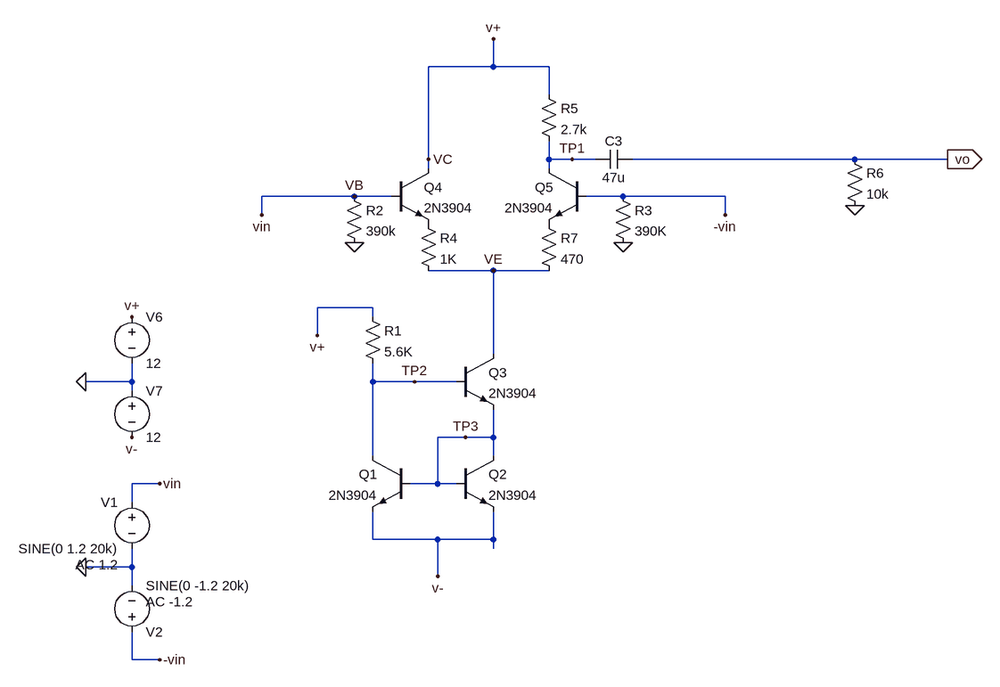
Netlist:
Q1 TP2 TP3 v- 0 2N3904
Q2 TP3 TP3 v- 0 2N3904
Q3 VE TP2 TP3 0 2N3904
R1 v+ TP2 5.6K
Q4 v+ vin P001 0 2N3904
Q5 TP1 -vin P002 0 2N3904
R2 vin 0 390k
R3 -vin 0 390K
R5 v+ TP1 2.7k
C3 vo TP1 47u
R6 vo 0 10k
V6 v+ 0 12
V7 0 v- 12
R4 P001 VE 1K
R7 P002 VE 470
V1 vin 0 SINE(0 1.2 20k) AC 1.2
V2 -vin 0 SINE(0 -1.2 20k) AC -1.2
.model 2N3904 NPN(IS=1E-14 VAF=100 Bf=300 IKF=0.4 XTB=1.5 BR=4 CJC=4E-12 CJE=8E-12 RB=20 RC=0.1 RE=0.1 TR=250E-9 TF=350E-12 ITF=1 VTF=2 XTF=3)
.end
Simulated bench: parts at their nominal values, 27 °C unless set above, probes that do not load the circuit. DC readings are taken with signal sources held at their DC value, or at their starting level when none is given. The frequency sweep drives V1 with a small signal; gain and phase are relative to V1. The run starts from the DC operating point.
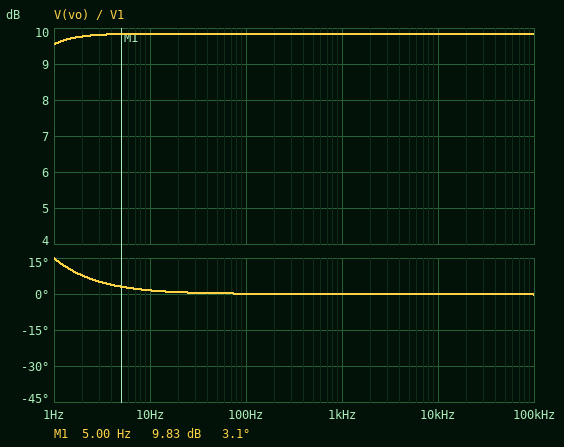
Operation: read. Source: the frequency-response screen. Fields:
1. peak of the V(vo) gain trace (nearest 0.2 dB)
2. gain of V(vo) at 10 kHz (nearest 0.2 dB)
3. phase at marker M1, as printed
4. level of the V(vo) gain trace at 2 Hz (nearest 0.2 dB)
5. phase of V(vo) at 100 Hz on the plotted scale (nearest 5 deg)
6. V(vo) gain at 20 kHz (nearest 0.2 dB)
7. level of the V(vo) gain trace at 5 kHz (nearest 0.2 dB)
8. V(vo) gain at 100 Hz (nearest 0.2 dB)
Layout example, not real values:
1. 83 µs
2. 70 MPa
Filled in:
1. 9.8 dB
2. 9.8 dB
3. 3.1 deg
4. 9.8 dB
5. 0 deg
6. 9.8 dB
7. 9.8 dB
8. 9.8 dB
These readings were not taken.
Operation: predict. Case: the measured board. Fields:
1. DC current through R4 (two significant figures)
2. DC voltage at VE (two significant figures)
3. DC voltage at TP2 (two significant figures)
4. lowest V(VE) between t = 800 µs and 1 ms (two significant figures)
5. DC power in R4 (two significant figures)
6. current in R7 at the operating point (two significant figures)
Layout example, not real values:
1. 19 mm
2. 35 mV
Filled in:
1. 1.3 mA
2. -2.0 V
3. -11 V
4. -2.4 V
5. 1.7 mW
6. 2.7 mA
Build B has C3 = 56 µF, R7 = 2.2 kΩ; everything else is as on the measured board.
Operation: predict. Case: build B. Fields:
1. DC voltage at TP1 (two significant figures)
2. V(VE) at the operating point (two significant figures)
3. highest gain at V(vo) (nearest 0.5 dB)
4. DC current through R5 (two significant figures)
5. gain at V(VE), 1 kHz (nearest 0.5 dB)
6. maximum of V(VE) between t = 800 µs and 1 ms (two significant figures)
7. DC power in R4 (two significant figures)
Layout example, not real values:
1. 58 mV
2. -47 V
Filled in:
1. 8.6 V
2. -3.4 V
3. 3.0 dB
4. 1.3 mA
5. -10.0 dB
6. -3.0 V
7. 7.6 mW
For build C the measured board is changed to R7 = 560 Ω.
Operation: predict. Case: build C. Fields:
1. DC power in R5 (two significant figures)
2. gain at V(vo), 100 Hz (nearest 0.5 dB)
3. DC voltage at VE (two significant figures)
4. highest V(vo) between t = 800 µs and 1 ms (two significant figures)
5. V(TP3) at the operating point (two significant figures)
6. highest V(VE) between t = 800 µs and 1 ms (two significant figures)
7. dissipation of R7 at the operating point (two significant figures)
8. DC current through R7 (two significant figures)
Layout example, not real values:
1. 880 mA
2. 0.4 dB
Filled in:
1. 18 mW
2. 9.5 dB
3. -2.1 V
4. 3.2 V
5. -11 V
6. -1.7 V
7. 3.7 mW
8. 2.6 mA
